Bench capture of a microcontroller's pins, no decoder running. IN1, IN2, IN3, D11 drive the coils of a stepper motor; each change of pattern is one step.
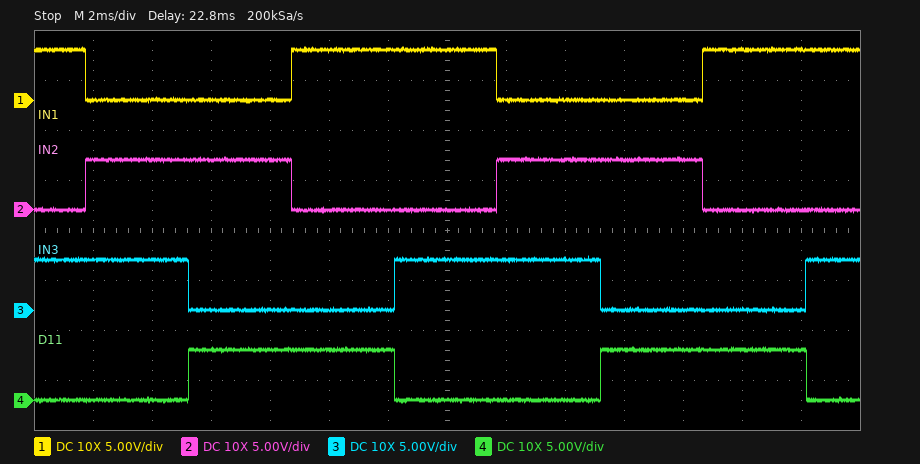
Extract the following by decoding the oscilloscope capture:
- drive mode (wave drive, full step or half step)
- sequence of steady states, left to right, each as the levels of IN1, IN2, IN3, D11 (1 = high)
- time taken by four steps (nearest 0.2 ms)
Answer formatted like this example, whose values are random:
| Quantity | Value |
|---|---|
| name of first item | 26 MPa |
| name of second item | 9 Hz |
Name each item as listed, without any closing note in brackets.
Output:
| Quantity | Value |
|---|---|
| drive mode | full step |
| sequence of steady states, left to right, each as the levels of IN1, IN2, IN3, D11 | 1010 0110 0101 1001 1010 0110 0101 1001 1010 |
| time taken by four steps | 14.0 ms |
